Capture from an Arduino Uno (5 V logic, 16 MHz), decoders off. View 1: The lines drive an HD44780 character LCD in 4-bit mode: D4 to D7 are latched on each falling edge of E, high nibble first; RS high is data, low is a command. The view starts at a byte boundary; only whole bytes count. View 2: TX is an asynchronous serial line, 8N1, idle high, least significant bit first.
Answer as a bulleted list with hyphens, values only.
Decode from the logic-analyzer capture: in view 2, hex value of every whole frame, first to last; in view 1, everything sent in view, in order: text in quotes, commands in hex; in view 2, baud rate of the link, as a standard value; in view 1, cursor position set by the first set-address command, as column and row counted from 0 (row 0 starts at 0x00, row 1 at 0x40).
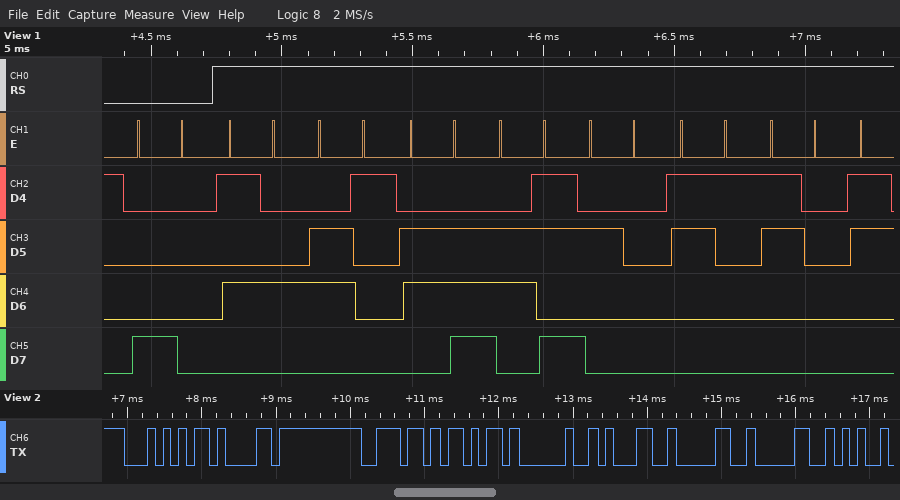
- 54 61 6E 6B 20 31 30 30
- 0x80 "Tank 10"
- 9600 baud
- column 0, row 0
